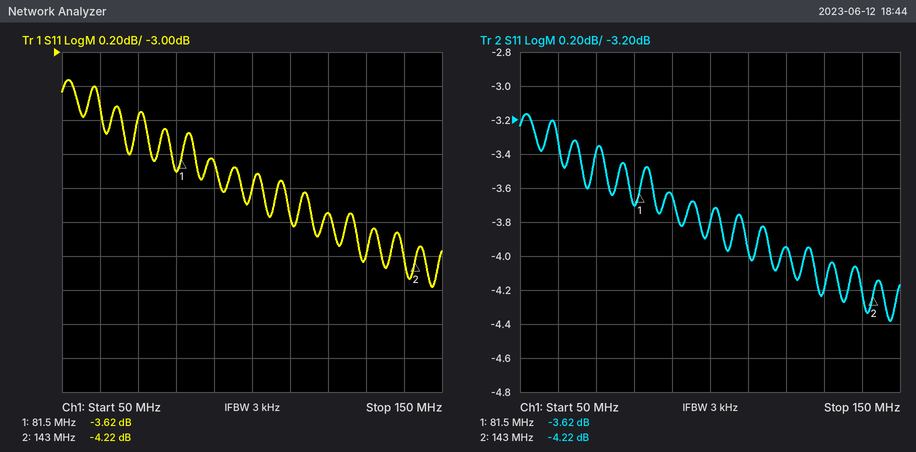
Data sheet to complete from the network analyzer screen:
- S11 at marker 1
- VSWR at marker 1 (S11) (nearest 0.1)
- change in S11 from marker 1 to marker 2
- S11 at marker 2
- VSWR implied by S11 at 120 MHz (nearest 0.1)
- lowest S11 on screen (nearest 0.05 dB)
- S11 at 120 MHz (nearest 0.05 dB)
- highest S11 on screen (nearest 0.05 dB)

-3.62 dB
4.9
-0.60 dB
-4.22 dB
4.5
-4.40 dB
-3.95 dB
-3.15 dB
